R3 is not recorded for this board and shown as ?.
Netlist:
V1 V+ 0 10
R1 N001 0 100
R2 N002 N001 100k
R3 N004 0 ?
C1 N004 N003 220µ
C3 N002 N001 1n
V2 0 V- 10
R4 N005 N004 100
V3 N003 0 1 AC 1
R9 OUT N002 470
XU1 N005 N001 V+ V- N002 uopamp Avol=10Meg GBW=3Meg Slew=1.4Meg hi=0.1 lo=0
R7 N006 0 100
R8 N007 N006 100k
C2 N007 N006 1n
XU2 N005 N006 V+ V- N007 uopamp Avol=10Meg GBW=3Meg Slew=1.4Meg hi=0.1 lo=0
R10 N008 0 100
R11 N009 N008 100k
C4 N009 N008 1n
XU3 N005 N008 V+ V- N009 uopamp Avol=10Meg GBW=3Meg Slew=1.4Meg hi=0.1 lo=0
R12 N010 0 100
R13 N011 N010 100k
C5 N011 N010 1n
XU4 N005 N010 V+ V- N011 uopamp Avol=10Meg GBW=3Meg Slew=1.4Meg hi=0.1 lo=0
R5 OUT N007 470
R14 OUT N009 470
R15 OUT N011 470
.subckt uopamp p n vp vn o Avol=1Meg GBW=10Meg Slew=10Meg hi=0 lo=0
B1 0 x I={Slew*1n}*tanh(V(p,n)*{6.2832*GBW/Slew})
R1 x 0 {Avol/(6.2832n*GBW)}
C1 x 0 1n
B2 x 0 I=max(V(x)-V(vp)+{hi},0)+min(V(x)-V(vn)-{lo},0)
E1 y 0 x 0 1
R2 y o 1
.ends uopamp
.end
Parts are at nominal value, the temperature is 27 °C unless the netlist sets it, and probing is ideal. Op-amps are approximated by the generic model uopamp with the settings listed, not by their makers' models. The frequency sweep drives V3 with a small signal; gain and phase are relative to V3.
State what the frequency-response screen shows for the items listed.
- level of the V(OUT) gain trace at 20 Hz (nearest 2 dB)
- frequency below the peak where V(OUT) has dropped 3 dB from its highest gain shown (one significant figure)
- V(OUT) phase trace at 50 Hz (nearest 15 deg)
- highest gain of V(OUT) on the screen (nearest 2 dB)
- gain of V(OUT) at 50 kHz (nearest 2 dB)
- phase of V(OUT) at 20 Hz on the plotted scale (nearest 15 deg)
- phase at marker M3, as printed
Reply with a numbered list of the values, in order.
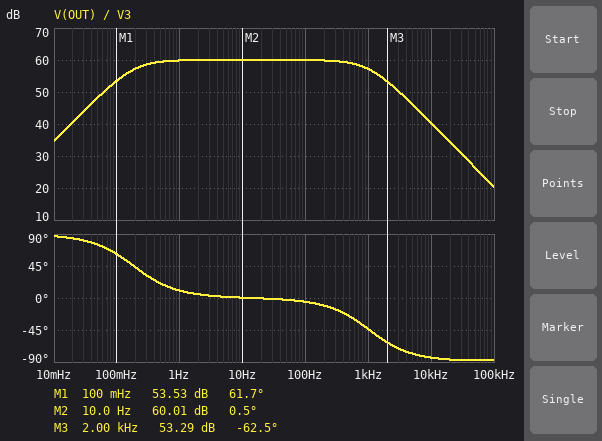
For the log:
1. 60 dB
2. 200 mHz
3. 0 deg
4. 60 dB
5. 26 dB
6. 0 deg
7. -62.5 deg
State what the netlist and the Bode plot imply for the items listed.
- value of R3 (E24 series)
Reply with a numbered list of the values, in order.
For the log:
1. 3.9 kΩ
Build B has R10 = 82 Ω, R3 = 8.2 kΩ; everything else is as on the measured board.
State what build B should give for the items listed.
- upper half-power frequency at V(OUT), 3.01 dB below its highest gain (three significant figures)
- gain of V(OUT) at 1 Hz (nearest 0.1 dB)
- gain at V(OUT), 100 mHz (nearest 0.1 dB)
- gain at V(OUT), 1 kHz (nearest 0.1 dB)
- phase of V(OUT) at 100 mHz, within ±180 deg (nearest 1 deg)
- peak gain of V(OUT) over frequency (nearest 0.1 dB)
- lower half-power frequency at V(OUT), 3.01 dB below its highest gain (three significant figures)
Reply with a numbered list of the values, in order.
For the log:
1. 1.02 kHz
2. 60.4 dB
3. 58.0 dB
4. 57.5 dB
5. 41 deg
6. 60.5 dB
7. 88.2 mHz
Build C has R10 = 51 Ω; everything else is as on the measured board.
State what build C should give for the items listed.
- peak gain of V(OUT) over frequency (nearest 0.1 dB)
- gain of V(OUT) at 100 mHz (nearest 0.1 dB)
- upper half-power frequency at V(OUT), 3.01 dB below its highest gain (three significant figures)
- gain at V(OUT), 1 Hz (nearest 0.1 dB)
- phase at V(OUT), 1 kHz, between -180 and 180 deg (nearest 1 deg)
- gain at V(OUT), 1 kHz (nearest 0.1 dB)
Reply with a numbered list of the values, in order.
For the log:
1. 61.9 dB
2. 55.4 dB
3. 920 Hz
4. 61.7 dB
5. -47 deg
6. 58.5 dB
